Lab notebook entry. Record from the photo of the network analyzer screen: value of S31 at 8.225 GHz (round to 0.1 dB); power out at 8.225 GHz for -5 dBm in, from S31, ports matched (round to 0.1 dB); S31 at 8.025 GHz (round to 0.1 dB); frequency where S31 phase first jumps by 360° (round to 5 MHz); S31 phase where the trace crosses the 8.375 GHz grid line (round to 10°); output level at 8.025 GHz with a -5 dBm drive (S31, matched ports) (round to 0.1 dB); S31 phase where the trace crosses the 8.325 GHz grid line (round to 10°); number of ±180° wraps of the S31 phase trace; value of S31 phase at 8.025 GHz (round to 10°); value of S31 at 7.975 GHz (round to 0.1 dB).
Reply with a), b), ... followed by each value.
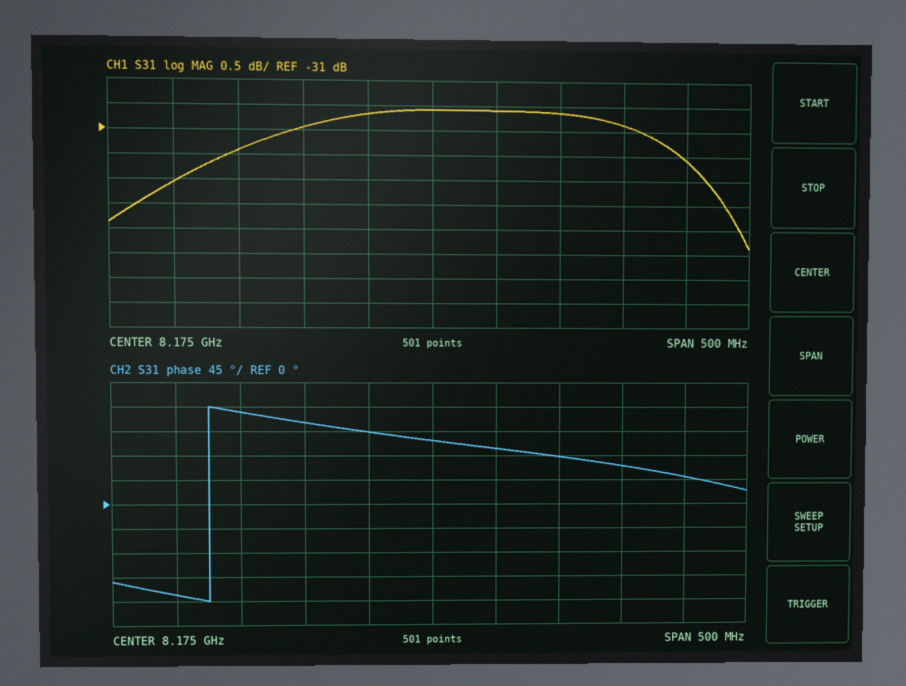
a) -30.6 dB
b) -35.6 dBm
c) -31.4 dB
d) 8.000 GHz
e) 50°
f) -36.4 dBm
g) 70°
h) 1
i) 170°
j) -32.1 dB
